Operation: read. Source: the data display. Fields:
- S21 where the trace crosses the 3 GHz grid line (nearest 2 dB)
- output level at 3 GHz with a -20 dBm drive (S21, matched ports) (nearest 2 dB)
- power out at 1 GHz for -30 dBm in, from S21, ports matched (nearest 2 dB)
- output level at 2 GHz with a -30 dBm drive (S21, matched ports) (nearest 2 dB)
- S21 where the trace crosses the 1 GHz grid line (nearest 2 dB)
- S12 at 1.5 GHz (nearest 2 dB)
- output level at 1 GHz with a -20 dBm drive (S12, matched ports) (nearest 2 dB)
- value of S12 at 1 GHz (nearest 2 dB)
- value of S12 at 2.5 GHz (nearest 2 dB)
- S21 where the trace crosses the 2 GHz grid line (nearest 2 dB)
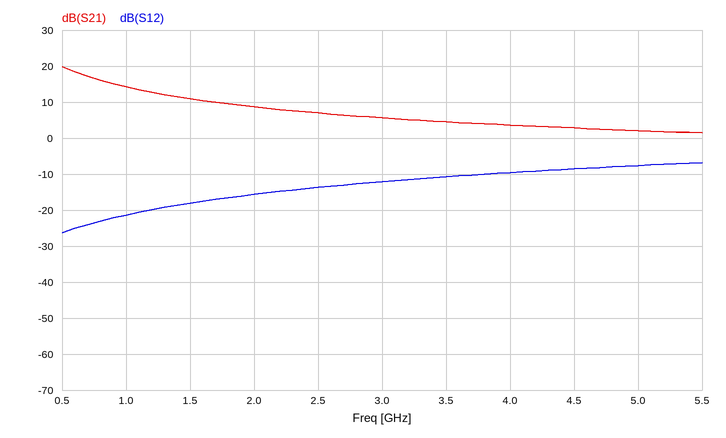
6 dB
-14 dBm
-16 dBm
-22 dBm
14 dB
-18 dB
-42 dBm
-22 dB
-14 dB
8 dB
